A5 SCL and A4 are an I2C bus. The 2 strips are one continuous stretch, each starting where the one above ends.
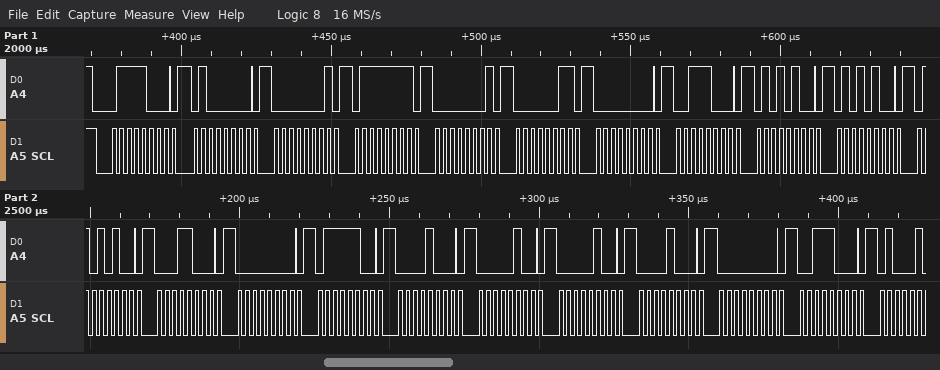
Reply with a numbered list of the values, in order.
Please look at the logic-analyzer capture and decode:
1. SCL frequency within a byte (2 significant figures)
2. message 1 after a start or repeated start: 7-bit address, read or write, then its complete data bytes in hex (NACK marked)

1. 400 kHz
2. 0x3C write: 40 01 7F 01 03 00 38 54 54 54 18 00 7C 08 04 04 08 00 38
